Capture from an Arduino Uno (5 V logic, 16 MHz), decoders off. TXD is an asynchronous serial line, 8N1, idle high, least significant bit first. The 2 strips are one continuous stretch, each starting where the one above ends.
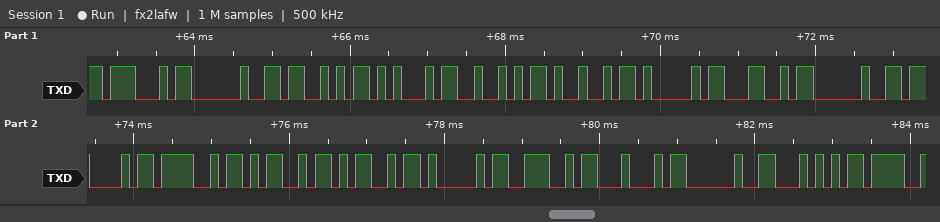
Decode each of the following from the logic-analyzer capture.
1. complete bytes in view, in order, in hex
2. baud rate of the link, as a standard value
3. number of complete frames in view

47 20 53 45 52 49 41 4C 20 43 4F 4D 4D 41 4E 44 20 54
9600 baud
18
